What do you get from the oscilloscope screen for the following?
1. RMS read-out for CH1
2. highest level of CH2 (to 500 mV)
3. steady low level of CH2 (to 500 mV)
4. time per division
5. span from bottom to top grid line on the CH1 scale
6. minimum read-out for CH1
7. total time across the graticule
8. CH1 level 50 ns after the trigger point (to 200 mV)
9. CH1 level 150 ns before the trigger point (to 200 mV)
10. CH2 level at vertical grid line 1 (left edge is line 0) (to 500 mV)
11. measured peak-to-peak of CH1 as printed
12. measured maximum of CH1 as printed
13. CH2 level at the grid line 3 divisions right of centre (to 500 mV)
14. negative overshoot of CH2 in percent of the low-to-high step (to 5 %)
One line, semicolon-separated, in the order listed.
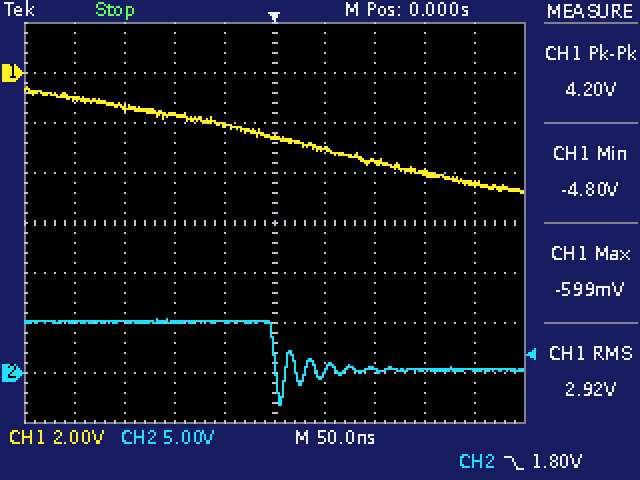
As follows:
2.92 V; 5.5 V; 500 mV; 50 ns; 16 V; -4.80 V; 500 ns; -3.0 V; -1.4 V; 5.0 V; 4.20 V; -599 mV; 500 mV; 75 %
